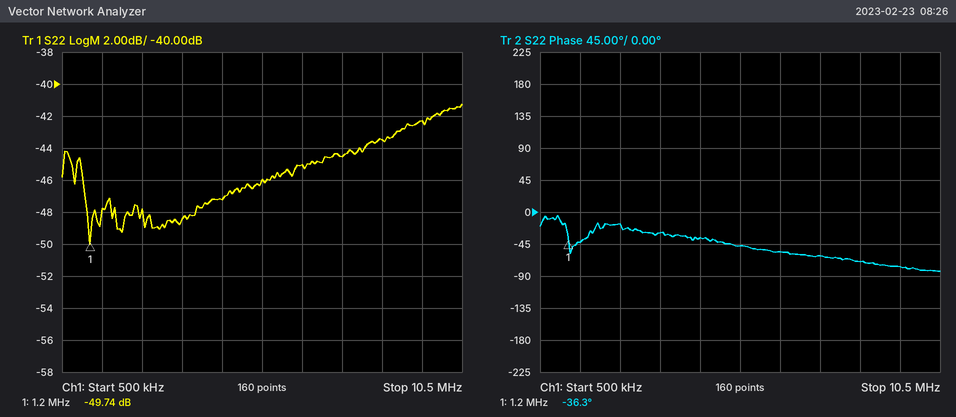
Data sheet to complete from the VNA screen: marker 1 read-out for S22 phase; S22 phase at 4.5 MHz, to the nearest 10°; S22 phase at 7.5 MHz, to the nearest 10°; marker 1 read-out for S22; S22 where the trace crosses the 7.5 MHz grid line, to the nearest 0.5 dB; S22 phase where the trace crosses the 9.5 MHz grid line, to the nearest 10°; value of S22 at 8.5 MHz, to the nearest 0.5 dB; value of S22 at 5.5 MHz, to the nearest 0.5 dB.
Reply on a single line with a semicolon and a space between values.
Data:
-36.3°; -40°; -60°; -49.74 dB; -44.5 dB; -80°; -43.5 dB; -46.0 dB
